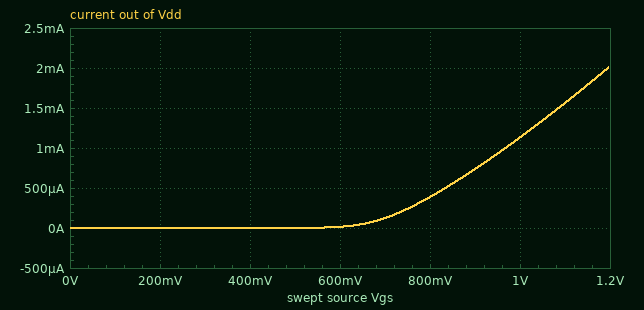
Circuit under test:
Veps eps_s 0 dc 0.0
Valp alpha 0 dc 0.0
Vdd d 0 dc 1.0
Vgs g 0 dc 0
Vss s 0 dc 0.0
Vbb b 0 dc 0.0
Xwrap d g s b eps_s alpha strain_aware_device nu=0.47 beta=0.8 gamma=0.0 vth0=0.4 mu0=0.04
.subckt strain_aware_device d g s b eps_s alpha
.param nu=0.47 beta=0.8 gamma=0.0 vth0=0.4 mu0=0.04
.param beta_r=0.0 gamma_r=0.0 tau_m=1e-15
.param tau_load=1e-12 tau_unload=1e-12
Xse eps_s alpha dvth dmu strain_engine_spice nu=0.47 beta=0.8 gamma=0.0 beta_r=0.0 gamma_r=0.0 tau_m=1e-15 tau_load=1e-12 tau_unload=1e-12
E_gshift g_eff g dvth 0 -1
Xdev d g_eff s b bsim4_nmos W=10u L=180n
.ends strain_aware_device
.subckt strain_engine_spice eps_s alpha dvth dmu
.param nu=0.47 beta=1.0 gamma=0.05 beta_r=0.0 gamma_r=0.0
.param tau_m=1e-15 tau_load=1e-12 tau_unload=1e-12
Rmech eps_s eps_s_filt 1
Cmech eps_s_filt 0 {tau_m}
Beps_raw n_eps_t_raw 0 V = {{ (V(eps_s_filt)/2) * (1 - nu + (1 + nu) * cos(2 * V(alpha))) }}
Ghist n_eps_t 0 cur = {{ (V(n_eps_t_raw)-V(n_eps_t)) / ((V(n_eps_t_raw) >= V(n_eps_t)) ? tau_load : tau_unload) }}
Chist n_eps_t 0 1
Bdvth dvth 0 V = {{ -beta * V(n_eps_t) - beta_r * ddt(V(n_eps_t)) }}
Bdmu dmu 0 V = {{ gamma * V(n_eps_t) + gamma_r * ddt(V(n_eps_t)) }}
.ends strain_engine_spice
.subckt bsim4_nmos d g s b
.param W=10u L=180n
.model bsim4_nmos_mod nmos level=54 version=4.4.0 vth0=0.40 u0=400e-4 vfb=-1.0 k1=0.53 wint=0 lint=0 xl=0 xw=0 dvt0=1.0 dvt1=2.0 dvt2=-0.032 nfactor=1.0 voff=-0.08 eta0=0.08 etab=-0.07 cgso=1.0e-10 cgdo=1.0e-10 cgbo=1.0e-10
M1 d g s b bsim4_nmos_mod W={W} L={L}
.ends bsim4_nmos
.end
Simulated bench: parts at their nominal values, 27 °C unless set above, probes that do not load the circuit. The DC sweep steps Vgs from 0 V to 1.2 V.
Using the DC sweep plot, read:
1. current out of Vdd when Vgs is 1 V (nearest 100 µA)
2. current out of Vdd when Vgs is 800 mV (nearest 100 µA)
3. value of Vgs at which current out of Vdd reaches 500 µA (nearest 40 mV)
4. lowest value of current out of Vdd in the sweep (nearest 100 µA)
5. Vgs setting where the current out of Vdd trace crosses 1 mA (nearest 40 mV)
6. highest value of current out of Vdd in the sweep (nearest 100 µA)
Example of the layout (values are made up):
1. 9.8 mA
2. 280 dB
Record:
1. 1.1 mA
2. 400 µA
3. 840 mV
4. 0 A
5. 960 mV
6. 2.0 mA
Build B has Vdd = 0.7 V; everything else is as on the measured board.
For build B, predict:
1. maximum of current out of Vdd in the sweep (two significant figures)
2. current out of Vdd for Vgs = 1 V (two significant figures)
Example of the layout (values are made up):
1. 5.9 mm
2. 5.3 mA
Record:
1. 1.9 mA
2. 1.0 mA
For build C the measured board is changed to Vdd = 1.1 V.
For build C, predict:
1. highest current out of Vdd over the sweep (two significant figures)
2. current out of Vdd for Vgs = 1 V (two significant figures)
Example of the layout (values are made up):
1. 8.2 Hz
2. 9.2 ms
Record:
1. 2.1 mA
2. 1.2 mA
